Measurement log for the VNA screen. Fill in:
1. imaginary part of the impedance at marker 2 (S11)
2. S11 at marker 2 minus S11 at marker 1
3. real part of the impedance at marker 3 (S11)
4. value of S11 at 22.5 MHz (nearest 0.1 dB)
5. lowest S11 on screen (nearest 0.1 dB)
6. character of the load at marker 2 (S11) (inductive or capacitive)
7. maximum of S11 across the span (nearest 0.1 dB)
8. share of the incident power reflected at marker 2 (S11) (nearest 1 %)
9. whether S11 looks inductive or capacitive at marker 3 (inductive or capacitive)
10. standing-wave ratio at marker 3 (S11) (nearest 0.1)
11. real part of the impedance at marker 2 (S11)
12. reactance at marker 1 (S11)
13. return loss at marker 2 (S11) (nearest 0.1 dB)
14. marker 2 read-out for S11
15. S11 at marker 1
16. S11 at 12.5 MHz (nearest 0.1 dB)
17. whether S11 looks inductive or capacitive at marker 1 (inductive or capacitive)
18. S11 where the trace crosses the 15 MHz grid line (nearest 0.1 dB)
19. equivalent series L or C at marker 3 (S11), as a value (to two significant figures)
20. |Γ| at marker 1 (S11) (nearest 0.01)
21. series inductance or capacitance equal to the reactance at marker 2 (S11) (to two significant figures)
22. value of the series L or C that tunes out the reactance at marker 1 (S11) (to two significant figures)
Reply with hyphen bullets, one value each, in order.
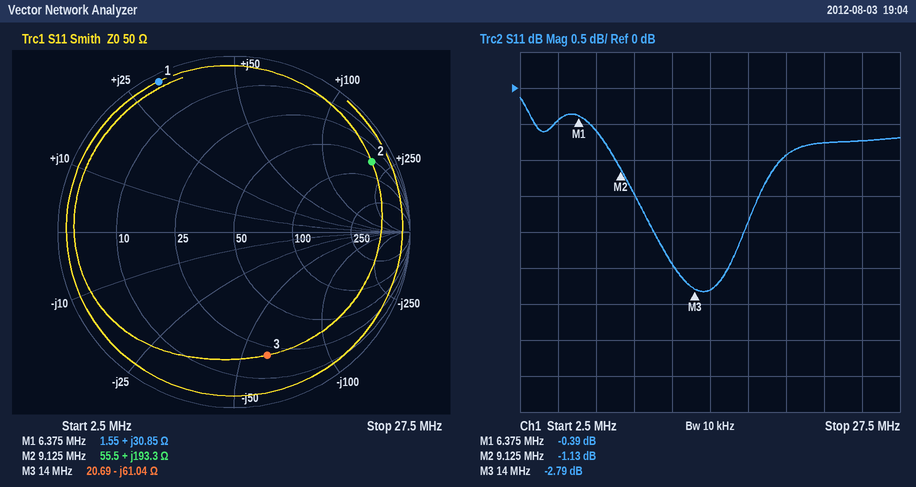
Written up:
- +193.3 Ω
- -0.74 dB
- 20.69 Ω
- -0.8 dB
- -2.8 dB
- inductive
- -0.1 dB
- 77 %
- capacitive
- 6.3
- 55.5 Ω
- +30.85 Ω
- 1.1 dB
- -1.13 dB
- -0.39 dB
- -2.4 dB
- inductive
- -2.8 dB
- 190 pF
- 0.96
- 3.4 µH
- 810 pF
